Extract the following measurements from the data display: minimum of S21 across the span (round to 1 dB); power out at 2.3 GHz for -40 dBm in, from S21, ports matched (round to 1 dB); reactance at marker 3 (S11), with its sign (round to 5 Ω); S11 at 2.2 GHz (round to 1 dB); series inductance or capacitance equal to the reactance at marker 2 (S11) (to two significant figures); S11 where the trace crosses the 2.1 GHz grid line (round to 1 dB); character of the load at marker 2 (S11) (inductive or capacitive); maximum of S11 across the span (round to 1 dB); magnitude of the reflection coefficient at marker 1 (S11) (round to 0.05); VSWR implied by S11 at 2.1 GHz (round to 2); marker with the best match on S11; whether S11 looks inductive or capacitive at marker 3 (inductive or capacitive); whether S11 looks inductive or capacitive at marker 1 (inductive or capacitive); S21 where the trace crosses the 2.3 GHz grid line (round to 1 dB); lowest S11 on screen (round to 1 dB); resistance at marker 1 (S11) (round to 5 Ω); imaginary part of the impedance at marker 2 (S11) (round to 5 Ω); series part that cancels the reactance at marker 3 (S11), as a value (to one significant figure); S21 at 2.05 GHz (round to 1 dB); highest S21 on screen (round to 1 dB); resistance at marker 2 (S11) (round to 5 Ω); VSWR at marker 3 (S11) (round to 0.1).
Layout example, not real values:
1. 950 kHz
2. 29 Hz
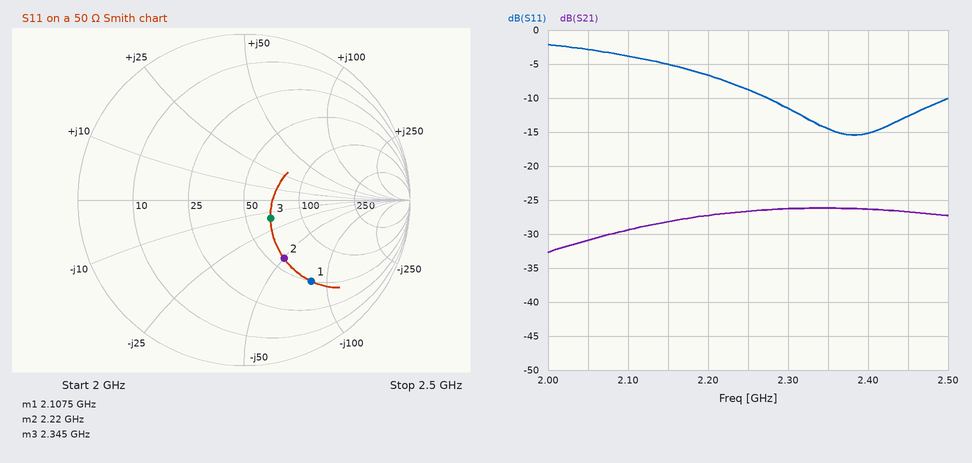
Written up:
1. -33 dB
2. -66 dBm
3. -15 Ω
4. -7 dB
5. 1.4 pF
6. -4 dB
7. capacitive
8. -2 dB
9. 0.65
10. 4
11. marker 3
12. capacitive
13. capacitive
14. -26 dB
15. -15 dB
16. 50 Ω
17. -50 Ω
18. 1 nH
19. -31 dB
20. -26 dB
21. 60 Ω
22. 1.5
